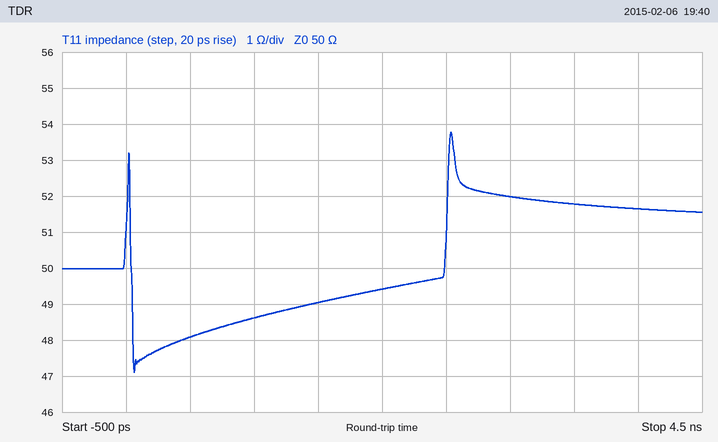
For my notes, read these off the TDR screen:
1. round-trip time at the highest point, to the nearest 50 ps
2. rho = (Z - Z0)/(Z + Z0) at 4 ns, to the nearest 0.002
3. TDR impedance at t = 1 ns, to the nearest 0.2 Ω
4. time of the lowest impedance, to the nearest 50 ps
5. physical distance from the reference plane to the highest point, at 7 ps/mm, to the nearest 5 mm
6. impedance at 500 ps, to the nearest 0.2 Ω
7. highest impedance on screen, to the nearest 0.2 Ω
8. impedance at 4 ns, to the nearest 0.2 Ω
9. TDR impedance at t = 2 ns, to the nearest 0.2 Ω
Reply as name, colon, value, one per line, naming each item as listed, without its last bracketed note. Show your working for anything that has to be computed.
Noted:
round-trip time at the highest point, to the nearest 50 ps: 2.55 ns
rho = (Z - Z0)/(Z + Z0) at 4 ns, to the nearest 0.002: (51.6 − 50)/(51.6 + 50) ≈ +0.016
TDR impedance at t = 1 ns, to the nearest 0.2 Ω: 48.6 Ω
time of the lowest impedance, to the nearest 50 ps: 50 ps
physical distance from the reference plane to the highest point, at 7 ps/mm, to the nearest 5 mm: 2.55 ns / 2 / 7 ps/mm ≈ 182 mm, so 180 mm to the nearest 5 mm
impedance at 500 ps, to the nearest 0.2 Ω: 48.0 Ω
highest impedance on screen, to the nearest 0.2 Ω: 53.8 Ω
impedance at 4 ns, to the nearest 0.2 Ω: 51.6 Ω
TDR impedance at t = 2 ns, to the nearest 0.2 Ω: 49.4 Ω
